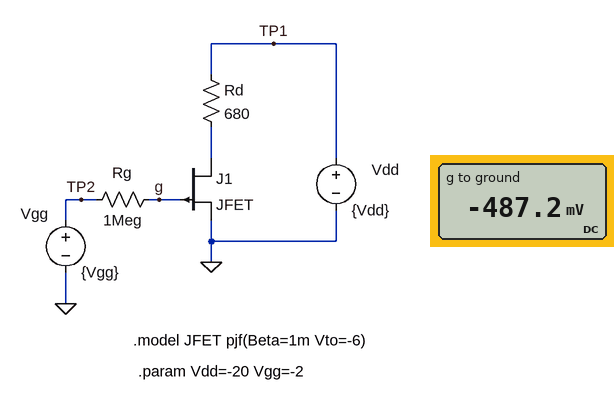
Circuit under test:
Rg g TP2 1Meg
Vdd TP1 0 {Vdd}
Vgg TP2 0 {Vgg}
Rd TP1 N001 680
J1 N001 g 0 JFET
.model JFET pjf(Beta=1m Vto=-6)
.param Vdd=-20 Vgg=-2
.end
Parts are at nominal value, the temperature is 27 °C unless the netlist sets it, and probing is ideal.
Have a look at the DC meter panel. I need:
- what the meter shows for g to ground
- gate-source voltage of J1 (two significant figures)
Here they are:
-487.2 mV
-490 mV
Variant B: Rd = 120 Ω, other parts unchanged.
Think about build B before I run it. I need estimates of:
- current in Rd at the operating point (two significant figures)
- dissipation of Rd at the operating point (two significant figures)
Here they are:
42 mA
210 mW
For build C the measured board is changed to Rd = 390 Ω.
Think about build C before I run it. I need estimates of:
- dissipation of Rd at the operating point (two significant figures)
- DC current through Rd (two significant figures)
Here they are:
600 mW
39 mA
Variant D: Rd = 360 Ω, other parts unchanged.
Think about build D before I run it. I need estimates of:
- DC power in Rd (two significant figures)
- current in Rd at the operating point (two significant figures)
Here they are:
600 mW
41 mA
